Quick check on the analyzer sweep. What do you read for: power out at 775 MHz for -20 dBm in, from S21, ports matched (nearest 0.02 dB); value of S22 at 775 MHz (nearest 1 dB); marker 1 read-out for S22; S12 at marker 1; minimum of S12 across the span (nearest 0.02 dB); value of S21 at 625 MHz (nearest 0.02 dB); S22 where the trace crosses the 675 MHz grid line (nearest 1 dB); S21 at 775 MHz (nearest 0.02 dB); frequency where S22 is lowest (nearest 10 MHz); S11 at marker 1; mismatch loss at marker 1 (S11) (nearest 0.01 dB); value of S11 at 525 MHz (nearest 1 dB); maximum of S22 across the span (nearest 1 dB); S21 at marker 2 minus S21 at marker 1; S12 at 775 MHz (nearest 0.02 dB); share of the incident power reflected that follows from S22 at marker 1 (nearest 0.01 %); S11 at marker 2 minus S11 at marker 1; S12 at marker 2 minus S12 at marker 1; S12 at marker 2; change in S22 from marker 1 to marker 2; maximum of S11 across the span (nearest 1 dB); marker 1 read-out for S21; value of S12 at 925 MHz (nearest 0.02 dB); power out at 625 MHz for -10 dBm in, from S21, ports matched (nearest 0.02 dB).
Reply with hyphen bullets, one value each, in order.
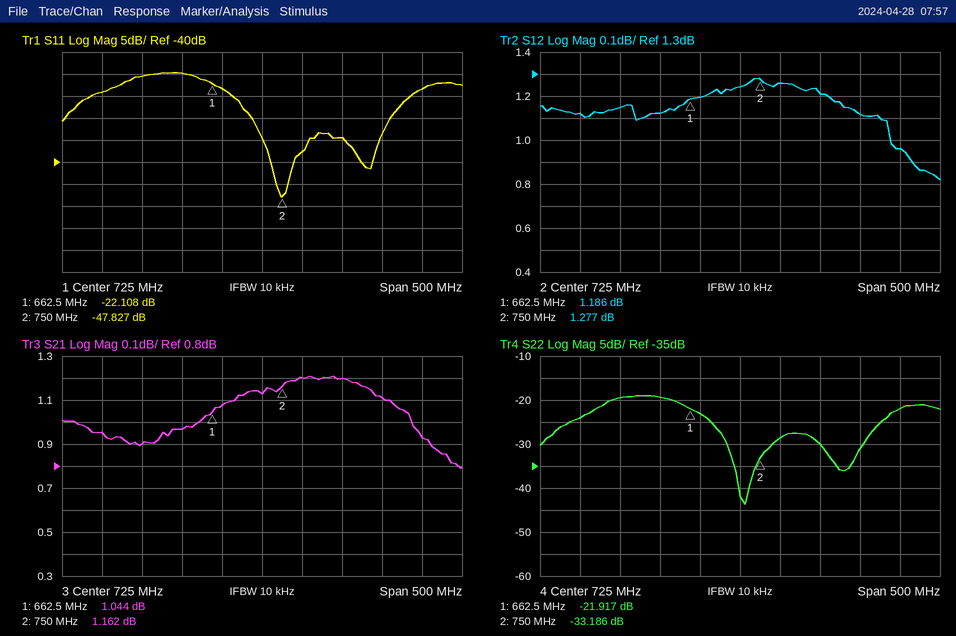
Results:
- -18.80 dBm
- -29 dB
- -21.917 dB
- 1.186 dB
- 0.82 dB
- 0.96 dB
- -23 dB
- 1.20 dB
- 730 MHz
- -22.108 dB
- 0.03 dB
- -24 dB
- -19 dB
- 0.118 dB
- 1.26 dB
- 0.64 %
- -25.719 dB
- 0.091 dB
- 1.277 dB
- -11.269 dB
- -20 dB
- 1.044 dB
- 0.96 dB
- -9.04 dBm
